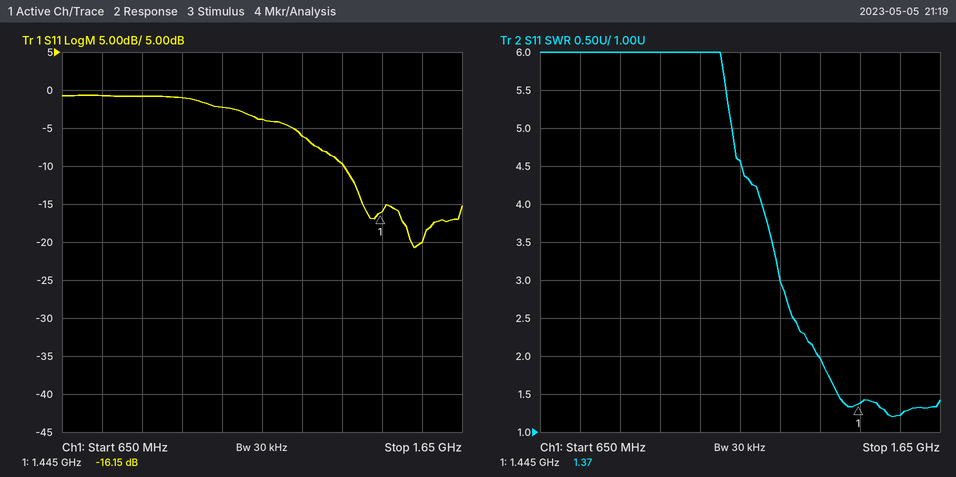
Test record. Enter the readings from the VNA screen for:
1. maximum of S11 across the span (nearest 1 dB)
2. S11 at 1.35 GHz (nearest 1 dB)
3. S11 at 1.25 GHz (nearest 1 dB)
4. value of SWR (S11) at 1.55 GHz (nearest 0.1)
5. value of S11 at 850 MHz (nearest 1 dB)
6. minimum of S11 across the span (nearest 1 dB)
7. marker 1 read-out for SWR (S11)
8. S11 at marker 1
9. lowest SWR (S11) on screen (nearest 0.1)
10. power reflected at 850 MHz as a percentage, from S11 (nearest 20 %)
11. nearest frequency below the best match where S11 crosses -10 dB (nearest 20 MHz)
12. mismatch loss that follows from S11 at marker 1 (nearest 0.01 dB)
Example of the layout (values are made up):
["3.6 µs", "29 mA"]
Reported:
["-1 dB", "-10 dB", "-6 dB", "1.2", "-1 dB", "-21 dB", "1.37", "-16.15 dB", "1.2", "80 %", "1.36 GHz", "0.11 dB"]
